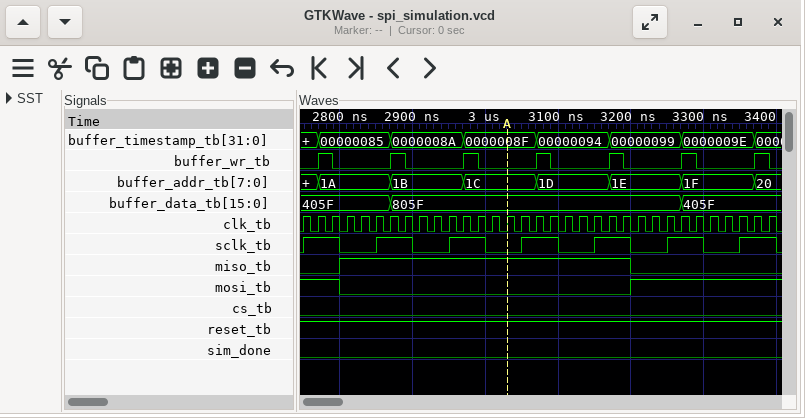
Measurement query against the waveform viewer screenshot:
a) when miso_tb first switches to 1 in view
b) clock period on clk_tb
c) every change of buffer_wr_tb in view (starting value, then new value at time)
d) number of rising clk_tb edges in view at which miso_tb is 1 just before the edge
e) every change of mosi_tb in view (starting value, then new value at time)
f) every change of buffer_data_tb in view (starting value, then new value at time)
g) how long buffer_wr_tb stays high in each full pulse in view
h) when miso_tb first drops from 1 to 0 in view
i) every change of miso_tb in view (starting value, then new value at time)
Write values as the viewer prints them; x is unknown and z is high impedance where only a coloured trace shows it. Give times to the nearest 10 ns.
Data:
2800 ns
20 ns
0, 1 at 2770 ns, 0 at 2790 ns, 1 at 2870 ns, 0 at 2890 ns, 1 at 2970 ns, 0 at 2990 ns, 1 at 3070 ns, 0 at 3090 ns, 1 at 3170 ns, 0 at 3190 ns, 1 at 3270 ns, 0 at 3290 ns, 1 at 3370 ns, 0 at 3390 ns
20
1, 0 at 2800 ns, 1 at 3200 ns
405F, 805F at 2870 ns, 405F at 3270 ns
20 ns, 20 ns, 20 ns, 20 ns, 20 ns, 20 ns, 20 ns
3200 ns
0, 1 at 2800 ns, 0 at 3200 ns
